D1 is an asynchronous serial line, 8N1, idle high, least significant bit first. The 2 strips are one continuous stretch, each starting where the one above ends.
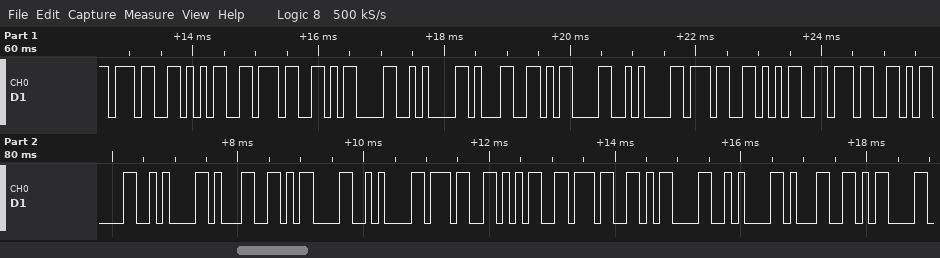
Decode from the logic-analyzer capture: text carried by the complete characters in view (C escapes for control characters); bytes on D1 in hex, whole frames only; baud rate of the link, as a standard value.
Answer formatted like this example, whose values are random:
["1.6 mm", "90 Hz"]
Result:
["\"757\\r\\n1\\r\\n757\\r\\n1\\r\\n757\\r\\n1\\r\"", "37 35 37 0D 0A 31 0D 0A 37 35 37 0D 0A 31 0D 0A 37 35 37 0D 0A 31 0D", "9600 baud"]
